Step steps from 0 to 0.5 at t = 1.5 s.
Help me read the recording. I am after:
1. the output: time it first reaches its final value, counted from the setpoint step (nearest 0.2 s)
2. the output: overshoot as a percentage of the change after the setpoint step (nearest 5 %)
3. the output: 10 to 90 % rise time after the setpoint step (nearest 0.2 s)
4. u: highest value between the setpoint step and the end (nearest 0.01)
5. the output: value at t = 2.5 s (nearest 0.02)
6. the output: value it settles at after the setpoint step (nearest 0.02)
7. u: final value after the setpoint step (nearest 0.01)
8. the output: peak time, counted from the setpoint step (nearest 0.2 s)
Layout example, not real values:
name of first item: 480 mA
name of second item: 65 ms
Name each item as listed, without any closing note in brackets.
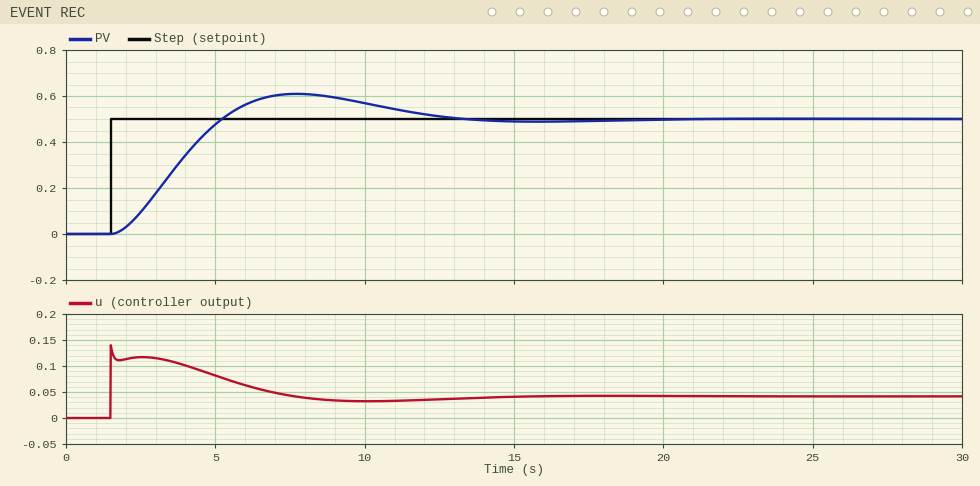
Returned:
the output: time it first reaches its final value, counted from the setpoint step: 3.8 s
the output: overshoot as a percentage of the change after the setpoint step: 20 %
the output: 10 to 90 % rise time after the setpoint step: 2.6 s
u: highest value between the setpoint step and the end: 0.14
the output: value at t = 2.5 s: 0.10
the output: value it settles at after the setpoint step: 0.50
u: final value after the setpoint step: 0.04
the output: peak time, counted from the setpoint step: 6.2 s
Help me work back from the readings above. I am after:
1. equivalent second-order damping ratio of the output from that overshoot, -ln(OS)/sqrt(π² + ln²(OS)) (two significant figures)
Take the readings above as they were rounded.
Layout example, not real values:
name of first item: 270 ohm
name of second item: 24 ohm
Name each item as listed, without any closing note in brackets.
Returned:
equivalent second-order damping ratio of the output from that overshoot, -ln(OS)/sqrt(π² + ln²(OS)): 0.46
